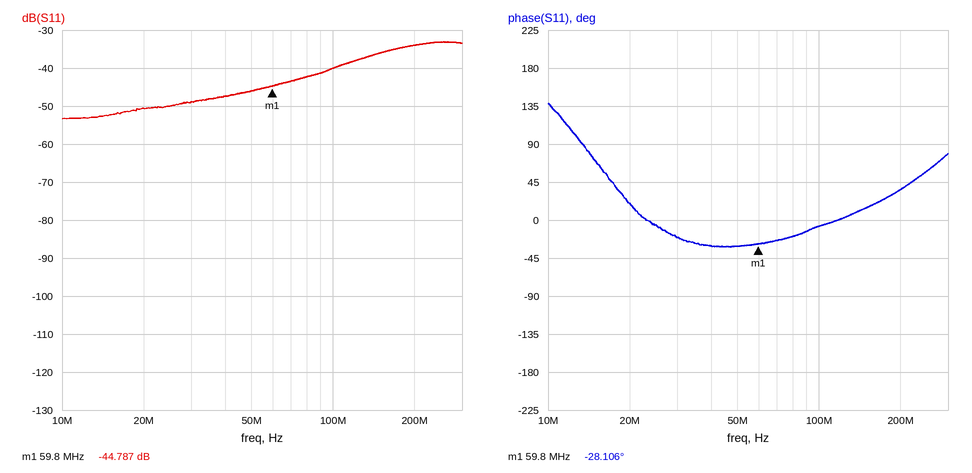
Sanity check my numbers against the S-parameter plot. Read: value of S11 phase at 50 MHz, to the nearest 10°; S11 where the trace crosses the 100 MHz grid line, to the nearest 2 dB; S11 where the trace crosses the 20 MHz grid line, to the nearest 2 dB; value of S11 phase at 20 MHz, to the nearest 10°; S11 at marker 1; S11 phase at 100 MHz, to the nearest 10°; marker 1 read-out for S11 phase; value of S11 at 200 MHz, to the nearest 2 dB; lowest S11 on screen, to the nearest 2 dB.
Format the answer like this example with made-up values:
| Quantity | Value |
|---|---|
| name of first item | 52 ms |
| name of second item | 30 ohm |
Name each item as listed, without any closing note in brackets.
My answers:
| Quantity | Value |
|---|---|
| value of S11 phase at 50 MHz, to the nearest 10° | -30° |
| S11 where the trace crosses the 100 MHz grid line, to the nearest 2 dB | -40 dB |
| S11 where the trace crosses the 20 MHz grid line, to the nearest 2 dB | -50 dB |
| value of S11 phase at 20 MHz, to the nearest 10° | 20° |
| S11 at marker 1 | -44.787 dB |
| S11 phase at 100 MHz, to the nearest 10° | -10° |
| marker 1 read-out for S11 phase | -28.106° |
| value of S11 at 200 MHz, to the nearest 2 dB | -34 dB |
| lowest S11 on screen, to the nearest 2 dB | -54 dB |
